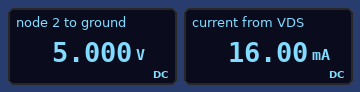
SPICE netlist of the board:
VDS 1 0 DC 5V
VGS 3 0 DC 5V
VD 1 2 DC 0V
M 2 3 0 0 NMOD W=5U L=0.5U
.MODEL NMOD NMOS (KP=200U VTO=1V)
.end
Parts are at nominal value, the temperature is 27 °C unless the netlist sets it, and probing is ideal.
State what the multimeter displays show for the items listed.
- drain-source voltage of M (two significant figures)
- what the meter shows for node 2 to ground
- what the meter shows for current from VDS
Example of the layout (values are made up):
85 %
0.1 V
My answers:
5.0 V
5.000 V
16.00 mA
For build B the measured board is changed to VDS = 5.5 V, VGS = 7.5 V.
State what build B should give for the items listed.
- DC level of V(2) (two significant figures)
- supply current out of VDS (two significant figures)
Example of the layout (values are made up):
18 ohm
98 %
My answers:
5.5 V
41 mA
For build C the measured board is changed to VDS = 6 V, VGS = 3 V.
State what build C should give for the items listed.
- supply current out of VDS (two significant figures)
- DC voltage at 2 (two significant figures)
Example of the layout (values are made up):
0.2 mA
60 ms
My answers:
4.0 mA
6.0 V
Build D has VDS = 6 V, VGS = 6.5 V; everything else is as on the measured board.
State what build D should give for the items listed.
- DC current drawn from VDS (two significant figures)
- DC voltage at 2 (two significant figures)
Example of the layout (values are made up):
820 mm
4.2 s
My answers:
30 mA
6.0 V
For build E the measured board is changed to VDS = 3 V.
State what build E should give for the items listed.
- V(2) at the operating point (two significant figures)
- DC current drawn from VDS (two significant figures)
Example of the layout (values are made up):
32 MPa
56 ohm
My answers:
3.0 V
15 mA
